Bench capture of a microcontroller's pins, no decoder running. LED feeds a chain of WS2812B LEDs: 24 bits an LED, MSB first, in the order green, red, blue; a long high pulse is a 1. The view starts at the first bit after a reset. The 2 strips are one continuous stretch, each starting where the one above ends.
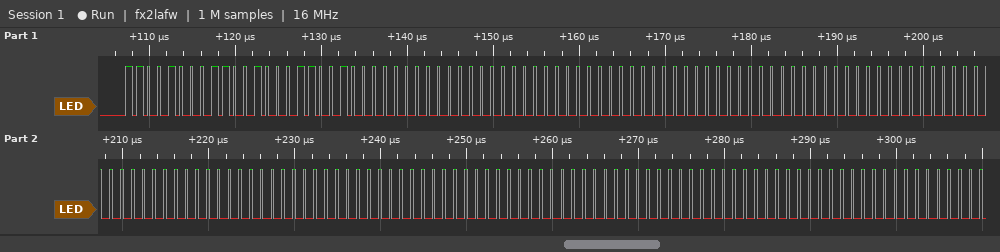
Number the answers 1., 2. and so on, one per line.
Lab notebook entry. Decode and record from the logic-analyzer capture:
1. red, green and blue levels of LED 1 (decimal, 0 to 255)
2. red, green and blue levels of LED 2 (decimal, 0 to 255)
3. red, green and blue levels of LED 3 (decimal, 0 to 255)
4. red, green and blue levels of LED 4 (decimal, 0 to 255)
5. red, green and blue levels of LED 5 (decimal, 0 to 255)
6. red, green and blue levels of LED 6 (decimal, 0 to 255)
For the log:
1. 200, 200, 200
2. 0, 0, 0
3. 0, 0, 0
4. 0, 0, 0
5. 0, 0, 0
6. 0, 0, 0
